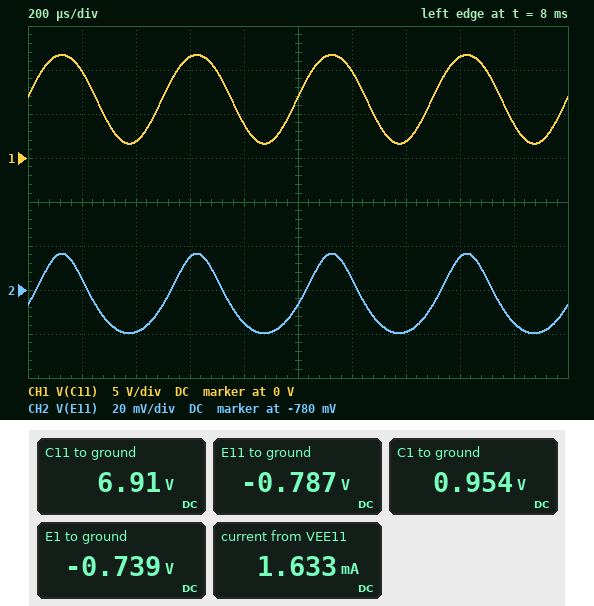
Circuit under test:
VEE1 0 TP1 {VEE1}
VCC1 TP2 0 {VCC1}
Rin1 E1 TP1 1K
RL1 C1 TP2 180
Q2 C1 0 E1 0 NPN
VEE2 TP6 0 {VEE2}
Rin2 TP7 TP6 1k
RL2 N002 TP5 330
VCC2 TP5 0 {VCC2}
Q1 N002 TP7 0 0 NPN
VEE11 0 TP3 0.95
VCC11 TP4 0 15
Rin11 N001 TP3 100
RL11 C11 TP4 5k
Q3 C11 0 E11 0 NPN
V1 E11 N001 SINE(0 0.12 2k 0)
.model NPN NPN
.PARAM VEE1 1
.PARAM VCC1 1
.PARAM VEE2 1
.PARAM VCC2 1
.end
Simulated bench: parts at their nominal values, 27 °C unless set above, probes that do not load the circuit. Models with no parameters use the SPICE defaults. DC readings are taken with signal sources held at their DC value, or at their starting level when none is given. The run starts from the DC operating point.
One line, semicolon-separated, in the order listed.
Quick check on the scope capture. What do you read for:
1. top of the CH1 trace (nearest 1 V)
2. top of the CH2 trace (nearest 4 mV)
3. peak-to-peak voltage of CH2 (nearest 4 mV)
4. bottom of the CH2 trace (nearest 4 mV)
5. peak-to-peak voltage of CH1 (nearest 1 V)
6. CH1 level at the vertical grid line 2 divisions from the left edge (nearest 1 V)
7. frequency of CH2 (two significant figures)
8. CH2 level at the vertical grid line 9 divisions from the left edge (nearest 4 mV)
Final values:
12 V; -764 mV; 36 mV; -800 mV; 10 V; 2 V; 2.0 kHz; -796 mV
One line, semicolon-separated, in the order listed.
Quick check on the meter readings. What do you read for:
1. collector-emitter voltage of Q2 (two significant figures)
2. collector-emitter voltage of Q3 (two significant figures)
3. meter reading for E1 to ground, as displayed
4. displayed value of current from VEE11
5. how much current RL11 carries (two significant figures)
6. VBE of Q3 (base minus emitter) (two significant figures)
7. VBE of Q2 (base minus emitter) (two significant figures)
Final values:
1.7 V; 7.7 V; -0.739 V; 1.633 mA; 1.6 mA; 790 mV; 740 mV
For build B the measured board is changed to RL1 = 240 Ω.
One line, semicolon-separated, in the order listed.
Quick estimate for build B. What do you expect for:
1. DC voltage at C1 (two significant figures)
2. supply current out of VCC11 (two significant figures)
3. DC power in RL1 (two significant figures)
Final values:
940 mV; 1.6 mA; 16 µW
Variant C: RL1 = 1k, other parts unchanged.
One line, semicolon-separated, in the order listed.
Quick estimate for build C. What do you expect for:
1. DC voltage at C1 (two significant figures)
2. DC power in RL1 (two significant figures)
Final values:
740 mV; 67 µW
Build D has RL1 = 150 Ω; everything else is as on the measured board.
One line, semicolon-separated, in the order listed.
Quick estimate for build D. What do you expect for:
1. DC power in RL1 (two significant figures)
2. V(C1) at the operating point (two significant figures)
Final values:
10 µW; 960 mV
